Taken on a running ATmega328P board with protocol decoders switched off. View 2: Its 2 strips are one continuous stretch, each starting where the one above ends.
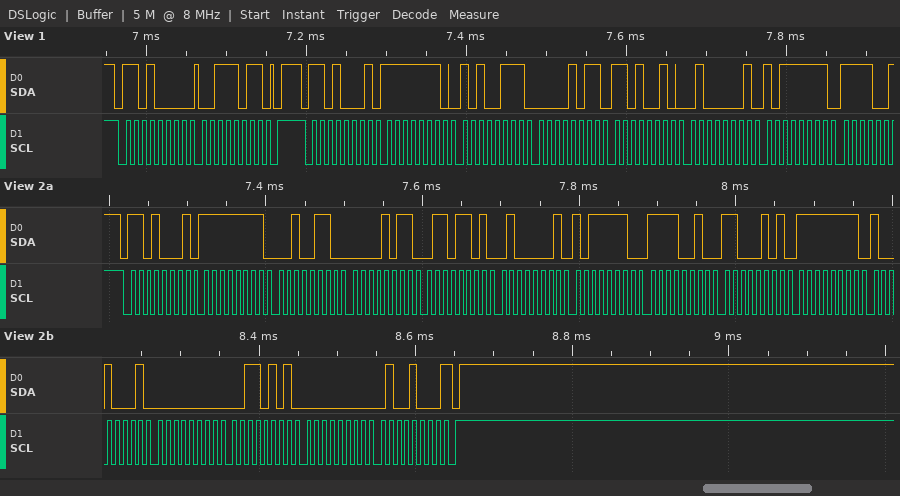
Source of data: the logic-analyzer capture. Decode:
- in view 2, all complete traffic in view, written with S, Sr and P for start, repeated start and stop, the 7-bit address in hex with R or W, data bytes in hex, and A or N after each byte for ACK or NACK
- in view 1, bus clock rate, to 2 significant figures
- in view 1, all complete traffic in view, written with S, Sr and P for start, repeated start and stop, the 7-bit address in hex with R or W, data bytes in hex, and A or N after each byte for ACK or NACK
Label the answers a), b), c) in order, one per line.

a) S 68R A FF A 26 A 0B A 6D A 41 A BE A F2 A C5 A FF A 91 A 00 A 35 A 00 A 48 N P
b) 100 kHz
c) S 68W A 3B A P S 68R A FE A A7 A 0B A D2 A 41 A BF A
